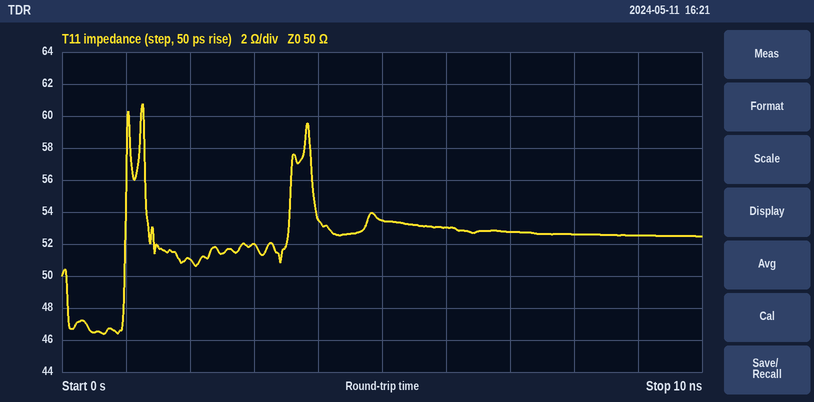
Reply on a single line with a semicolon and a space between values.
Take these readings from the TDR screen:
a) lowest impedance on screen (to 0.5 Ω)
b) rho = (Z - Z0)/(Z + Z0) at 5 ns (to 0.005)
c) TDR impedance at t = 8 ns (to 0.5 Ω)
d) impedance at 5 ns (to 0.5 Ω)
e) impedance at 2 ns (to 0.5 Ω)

46.5 Ω; +0.035; 52.5 Ω; 53.5 Ω; 51.0 Ω
